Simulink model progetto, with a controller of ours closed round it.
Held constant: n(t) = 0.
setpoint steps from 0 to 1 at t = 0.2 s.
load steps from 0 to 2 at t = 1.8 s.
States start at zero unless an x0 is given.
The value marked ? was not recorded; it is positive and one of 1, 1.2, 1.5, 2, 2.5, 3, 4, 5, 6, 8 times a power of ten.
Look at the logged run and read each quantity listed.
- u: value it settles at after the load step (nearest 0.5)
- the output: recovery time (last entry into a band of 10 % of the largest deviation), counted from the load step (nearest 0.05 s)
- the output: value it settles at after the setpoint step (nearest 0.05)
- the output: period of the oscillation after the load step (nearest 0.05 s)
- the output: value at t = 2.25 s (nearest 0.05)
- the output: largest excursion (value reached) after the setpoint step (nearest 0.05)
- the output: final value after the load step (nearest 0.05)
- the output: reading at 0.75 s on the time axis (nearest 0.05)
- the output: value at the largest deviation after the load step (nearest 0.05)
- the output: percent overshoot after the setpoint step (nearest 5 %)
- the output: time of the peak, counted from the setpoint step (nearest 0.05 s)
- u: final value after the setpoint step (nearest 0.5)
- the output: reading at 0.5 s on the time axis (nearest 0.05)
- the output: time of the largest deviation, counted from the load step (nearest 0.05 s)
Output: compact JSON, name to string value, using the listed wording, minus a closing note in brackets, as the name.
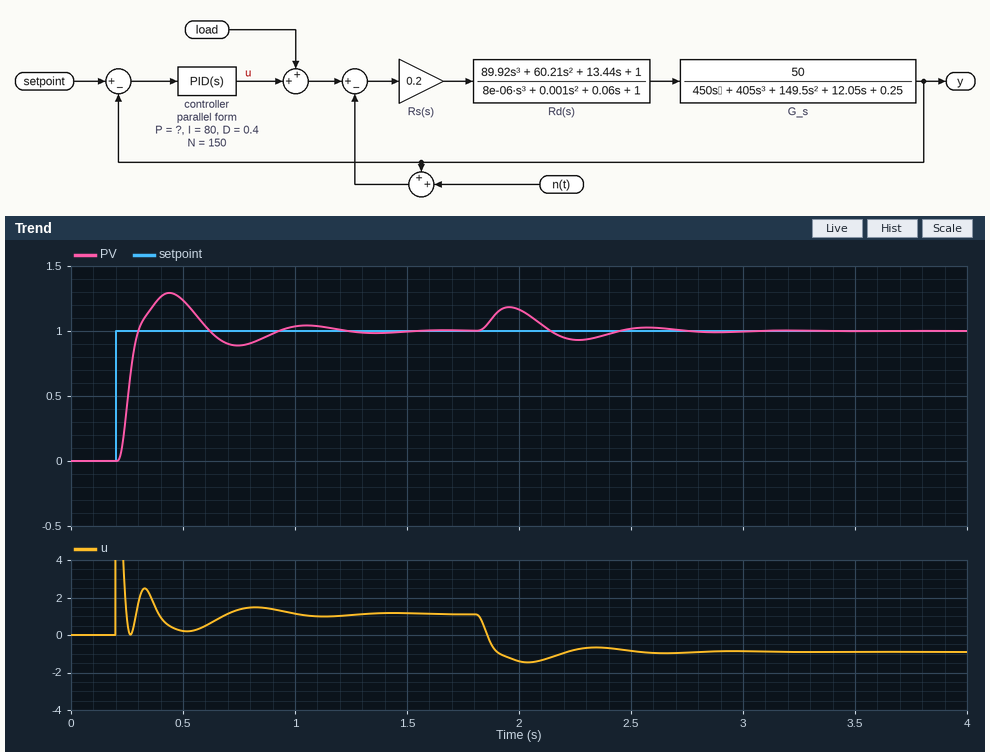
{"u: value it settles at after the load step": "-1.0", "the output: recovery time (last entry into a band of 10 % of the largest deviation), counted from the load step": "0.85 s", "the output: value it settles at after the setpoint step": "1.00", "the output: period of the oscillation after the load step": "0.60 s", "the output: value at t = 2.25 s": "0.95", "the output: largest excursion (value reached) after the setpoint step": "1.30", "the output: final value after the load step": "1.00", "the output: reading at 0.75 s on the time axis": "0.90", "the output: value at the largest deviation after the load step": "1.20", "the output: percent overshoot after the setpoint step": "30 %", "the output: time of the peak, counted from the setpoint step": "0.25 s", "u: final value after the setpoint step": "1.0", "the output: reading at 0.5 s on the time axis": "1.25", "the output: time of the largest deviation, counted from the load step": "0.15 s"}
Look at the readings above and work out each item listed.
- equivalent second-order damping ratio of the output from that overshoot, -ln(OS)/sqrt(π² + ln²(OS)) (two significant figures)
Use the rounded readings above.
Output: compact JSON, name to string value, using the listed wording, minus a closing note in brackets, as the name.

{"equivalent second-order damping ratio of the output from that overshoot, -ln(OS)/sqrt(π² + ln²(OS))": "0.36"}
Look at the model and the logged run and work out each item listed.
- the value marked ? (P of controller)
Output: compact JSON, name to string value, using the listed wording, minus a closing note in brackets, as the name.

{"the value marked ?": "6"}
